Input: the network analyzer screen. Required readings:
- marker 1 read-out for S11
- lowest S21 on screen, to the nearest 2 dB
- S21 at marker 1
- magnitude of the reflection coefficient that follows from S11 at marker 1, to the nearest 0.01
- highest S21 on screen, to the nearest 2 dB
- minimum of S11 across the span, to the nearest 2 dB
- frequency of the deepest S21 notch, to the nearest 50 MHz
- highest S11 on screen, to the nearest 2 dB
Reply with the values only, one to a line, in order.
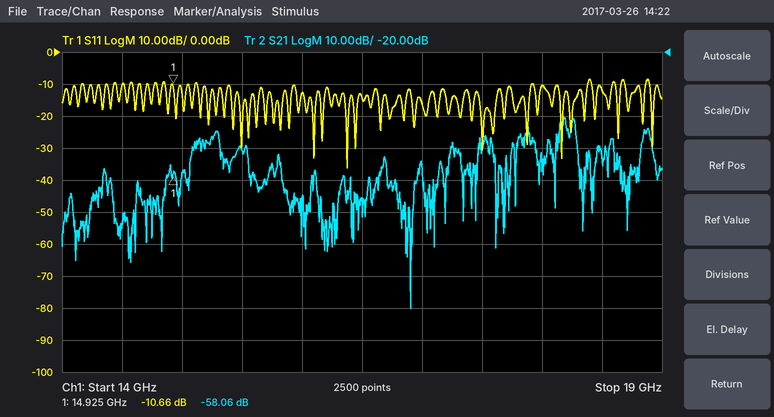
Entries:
-10.66 dB
-100 dB
-58.06 dB
0.29
-40 dB
-36 dB
16.90 GHz
-8 dB
